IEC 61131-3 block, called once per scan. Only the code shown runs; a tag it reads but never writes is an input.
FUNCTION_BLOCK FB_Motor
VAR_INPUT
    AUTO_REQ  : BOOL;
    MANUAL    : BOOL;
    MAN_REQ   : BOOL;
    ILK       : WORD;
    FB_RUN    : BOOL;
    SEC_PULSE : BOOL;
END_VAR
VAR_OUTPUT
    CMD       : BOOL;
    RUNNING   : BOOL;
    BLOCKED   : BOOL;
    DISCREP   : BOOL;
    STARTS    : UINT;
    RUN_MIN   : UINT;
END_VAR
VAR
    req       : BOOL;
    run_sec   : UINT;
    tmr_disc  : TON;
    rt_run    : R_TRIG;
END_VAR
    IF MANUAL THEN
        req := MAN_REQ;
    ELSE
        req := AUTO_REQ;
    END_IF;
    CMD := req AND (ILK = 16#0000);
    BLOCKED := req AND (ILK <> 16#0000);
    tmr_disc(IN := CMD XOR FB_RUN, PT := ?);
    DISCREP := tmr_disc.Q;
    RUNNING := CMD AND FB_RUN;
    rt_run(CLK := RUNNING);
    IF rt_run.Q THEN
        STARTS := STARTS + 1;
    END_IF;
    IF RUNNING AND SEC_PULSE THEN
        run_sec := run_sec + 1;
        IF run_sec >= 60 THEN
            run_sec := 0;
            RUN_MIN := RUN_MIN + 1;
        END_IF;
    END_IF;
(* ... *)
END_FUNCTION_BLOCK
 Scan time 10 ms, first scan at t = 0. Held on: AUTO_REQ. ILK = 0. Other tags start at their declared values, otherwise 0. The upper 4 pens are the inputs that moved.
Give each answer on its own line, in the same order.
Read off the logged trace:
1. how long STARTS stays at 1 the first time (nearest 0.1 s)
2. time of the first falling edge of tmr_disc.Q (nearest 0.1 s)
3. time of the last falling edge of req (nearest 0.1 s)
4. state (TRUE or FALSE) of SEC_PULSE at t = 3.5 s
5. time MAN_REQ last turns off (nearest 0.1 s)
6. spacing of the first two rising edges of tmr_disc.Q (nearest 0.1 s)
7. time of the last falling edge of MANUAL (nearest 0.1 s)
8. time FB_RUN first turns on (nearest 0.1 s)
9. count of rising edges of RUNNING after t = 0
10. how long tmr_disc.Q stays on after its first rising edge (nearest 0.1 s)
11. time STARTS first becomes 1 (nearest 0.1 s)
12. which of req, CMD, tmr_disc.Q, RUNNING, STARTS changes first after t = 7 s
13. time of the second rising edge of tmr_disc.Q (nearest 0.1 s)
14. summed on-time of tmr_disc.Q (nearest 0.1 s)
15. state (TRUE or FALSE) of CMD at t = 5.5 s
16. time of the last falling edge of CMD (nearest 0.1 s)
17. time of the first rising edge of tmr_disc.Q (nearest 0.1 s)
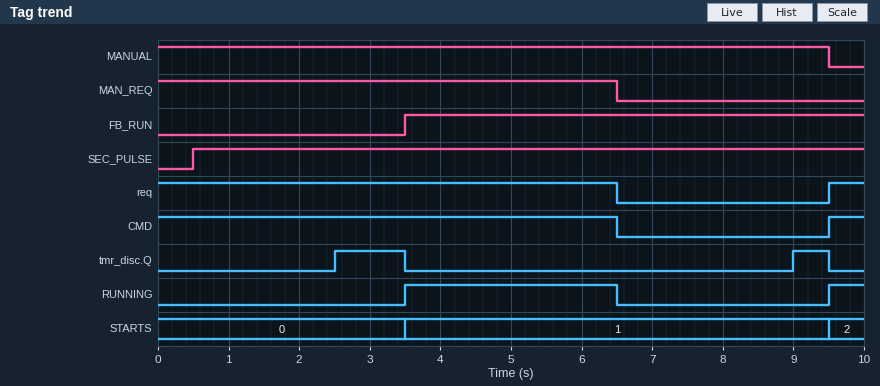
6.0 s
3.5 s
6.5 s
TRUE
6.5 s
6.5 s
9.5 s
3.5 s
2
1.0 s
3.5 s
tmr_disc.Q
9.0 s
1.5 s
TRUE
6.5 s
2.5 s
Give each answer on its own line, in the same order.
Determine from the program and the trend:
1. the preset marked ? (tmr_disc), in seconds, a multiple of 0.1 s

2.5 s
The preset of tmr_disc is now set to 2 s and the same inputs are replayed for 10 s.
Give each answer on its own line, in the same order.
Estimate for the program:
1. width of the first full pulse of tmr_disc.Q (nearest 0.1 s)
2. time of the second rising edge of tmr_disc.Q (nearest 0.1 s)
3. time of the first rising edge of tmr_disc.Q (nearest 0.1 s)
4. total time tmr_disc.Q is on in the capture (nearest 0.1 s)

1.5 s
8.5 s
2.0 s
2.5 s
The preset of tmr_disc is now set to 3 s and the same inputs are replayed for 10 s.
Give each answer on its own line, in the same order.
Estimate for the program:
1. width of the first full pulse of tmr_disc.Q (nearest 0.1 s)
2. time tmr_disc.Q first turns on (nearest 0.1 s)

0.5 s
3.0 s
